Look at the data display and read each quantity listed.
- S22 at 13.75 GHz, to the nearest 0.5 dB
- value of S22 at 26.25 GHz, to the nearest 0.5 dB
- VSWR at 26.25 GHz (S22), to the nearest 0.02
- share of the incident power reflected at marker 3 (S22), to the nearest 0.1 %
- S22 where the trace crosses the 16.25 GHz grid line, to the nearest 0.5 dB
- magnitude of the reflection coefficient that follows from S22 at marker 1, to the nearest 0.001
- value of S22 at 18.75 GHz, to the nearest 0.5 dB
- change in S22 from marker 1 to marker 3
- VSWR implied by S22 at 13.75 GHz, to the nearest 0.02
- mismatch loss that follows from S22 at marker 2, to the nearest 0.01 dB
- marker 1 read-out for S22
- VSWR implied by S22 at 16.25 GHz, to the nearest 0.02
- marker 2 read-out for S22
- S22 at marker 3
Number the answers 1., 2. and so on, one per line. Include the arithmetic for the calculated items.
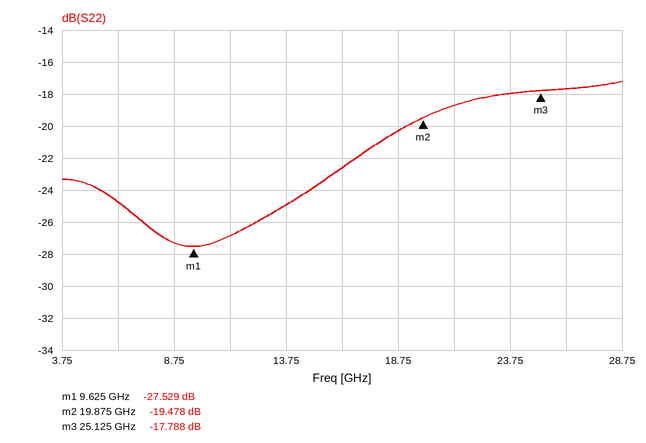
1. -25.0 dB
2. -17.5 dB
3. |Γ| = 10^(-17.5/20) = 0.1334; VSWR = (1 + 0.1334)/(1 − 0.1334) ≈ 1.31, so 1.30 to the nearest 0.02
4. 10^(-17.788/10) ≈ 1.7 %
5. -22.5 dB
6. 10^(-27.529/20) ≈ 0.042
7. -20.5 dB
8. -17.788 − (-27.529) = 9.741 dB
9. |Γ| = 10^(-25/20) = 0.0562; VSWR = (1 + 0.0562)/(1 − 0.0562) ≈ 1.12
10. −10 log10(1 − 10^(-19.478/10)) ≈ 0.05 dB
11. -27.529 dB
12. |Γ| = 10^(-22.5/20) = 0.0750; VSWR = (1 + 0.0750)/(1 − 0.0750) ≈ 1.16
13. -19.478 dB
14. -17.788 dB
